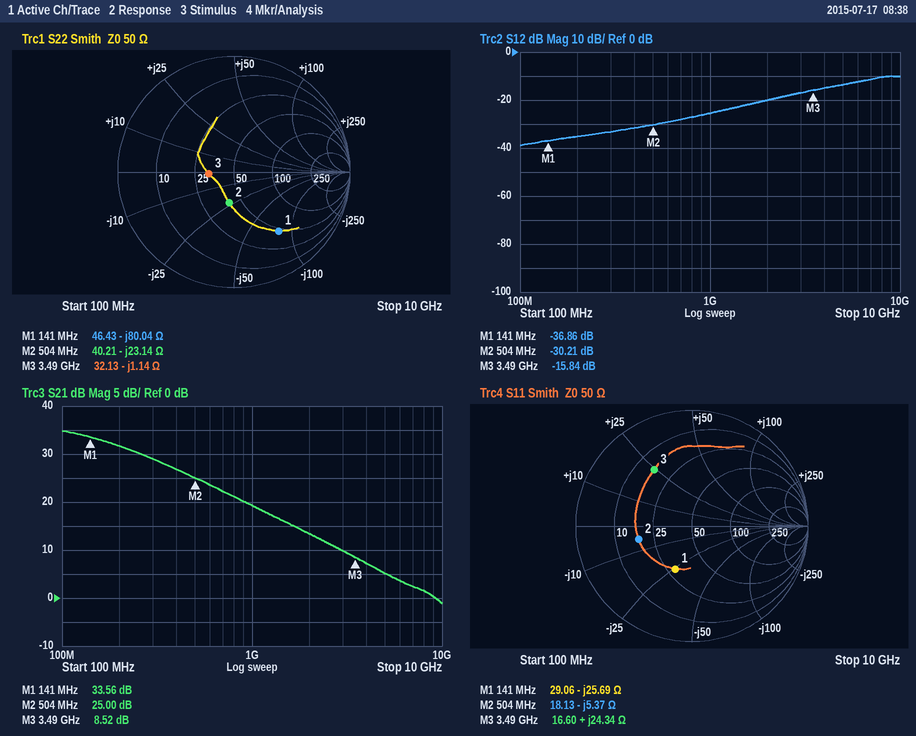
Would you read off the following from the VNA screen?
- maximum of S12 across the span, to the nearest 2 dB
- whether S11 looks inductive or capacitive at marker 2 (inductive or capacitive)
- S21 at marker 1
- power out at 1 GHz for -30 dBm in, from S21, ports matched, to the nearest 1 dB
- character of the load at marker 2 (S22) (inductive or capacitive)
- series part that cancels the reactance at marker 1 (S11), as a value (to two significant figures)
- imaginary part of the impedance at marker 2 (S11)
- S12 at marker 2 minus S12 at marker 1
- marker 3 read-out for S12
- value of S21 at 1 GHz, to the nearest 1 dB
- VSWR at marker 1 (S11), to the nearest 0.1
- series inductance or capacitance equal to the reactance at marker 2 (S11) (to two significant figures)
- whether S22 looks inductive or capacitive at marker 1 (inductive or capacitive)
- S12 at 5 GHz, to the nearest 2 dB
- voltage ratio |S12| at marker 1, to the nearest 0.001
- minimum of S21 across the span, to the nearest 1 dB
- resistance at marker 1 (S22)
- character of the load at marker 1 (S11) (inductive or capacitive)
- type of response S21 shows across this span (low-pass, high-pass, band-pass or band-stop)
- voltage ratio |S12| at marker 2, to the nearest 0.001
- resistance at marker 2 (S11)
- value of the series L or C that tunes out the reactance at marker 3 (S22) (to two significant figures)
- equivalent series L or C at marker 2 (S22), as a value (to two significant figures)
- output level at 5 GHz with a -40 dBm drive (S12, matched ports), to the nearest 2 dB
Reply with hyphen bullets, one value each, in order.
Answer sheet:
- -10 dB
- capacitive
- 33.56 dB
- -11 dBm
- capacitive
- 29 nH
- -5.37 Ω
- 6.65 dB
- -15.84 dB
- 19 dB
- 2.3
- 59 pF
- capacitive
- -14 dB
- 0.014
- -1 dB
- 46.43 Ω
- capacitive
- low-pass
- 0.031
- 18.13 Ω
- 52 pH
- 14 pF
- -54 dBm
